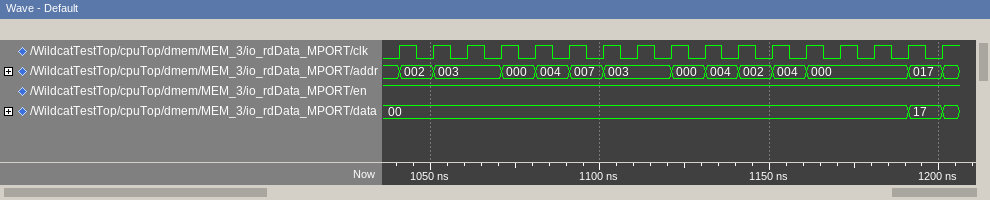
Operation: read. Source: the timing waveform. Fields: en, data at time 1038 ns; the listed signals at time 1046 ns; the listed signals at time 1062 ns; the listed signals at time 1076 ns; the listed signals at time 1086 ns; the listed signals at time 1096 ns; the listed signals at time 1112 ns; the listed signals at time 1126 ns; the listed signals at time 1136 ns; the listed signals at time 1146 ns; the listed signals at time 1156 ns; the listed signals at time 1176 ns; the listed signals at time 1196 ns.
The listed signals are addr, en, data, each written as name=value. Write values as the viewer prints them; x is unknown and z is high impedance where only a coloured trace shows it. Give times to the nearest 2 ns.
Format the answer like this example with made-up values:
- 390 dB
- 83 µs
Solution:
- en=1, data=00
- addr=002, en=1, data=00
- addr=003, en=1, data=00
- addr=000, en=1, data=00
- addr=004, en=1, data=00
- addr=007, en=1, data=00
- addr=003, en=1, data=00
- addr=000, en=1, data=00
- addr=004, en=1, data=00
- addr=002, en=1, data=00
- addr=004, en=1, data=00
- addr=000, en=1, data=00
- addr=017, en=1, data=17
